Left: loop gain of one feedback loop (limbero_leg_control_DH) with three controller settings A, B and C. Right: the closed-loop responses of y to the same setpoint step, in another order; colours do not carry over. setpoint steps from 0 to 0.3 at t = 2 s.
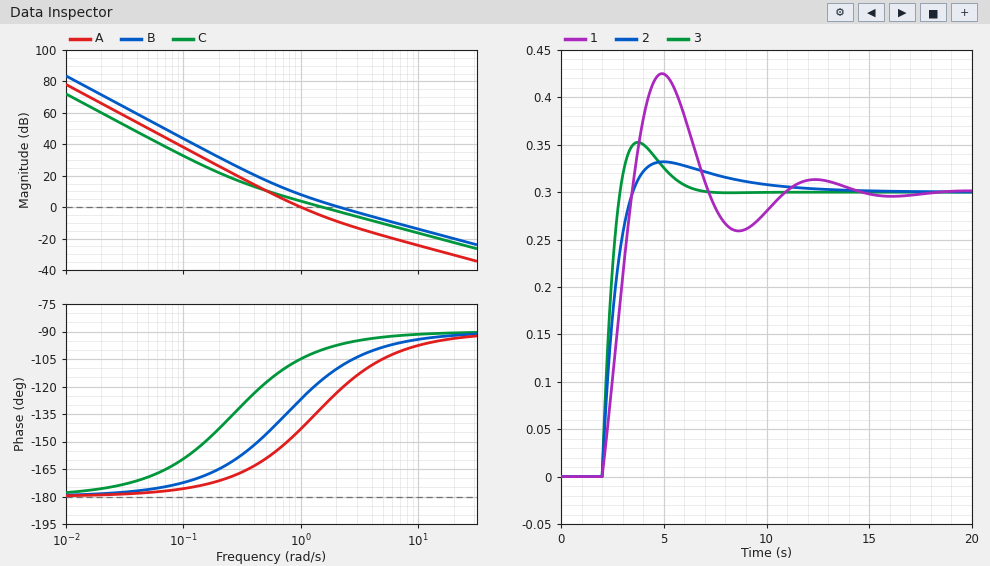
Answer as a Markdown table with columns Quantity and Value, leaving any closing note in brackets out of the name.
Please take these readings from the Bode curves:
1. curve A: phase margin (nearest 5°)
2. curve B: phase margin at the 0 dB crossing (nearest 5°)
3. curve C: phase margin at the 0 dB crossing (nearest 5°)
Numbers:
| Quantity | Value |
|---|---|
| curve A: phase margin | 35° |
| curve B: phase margin at the 0 dB crossing | 70° |
| curve C: phase margin at the 0 dB crossing | 80° |
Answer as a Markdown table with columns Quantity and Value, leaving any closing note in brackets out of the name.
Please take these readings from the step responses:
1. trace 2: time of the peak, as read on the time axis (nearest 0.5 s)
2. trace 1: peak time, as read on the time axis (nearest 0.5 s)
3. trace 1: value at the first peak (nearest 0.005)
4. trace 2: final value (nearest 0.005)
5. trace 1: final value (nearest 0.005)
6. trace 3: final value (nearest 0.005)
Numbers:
| Quantity | Value |
|---|---|
| trace 2: time of the peak, as read on the time axis | 5.0 s |
| trace 1: peak time, as read on the time axis | 5.0 s |
| trace 1: value at the first peak | 0.425 |
| trace 2: final value | 0.300 |
| trace 1: final value | 0.300 |
| trace 3: final value | 0.300 |
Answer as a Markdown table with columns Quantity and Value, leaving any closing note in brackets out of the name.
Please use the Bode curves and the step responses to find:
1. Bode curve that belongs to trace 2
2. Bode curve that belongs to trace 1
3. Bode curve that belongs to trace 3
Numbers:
| Quantity | Value |
|---|---|
| Bode curve that belongs to trace 2 | C |
| Bode curve that belongs to trace 1 | A |
| Bode curve that belongs to trace 3 | B |
